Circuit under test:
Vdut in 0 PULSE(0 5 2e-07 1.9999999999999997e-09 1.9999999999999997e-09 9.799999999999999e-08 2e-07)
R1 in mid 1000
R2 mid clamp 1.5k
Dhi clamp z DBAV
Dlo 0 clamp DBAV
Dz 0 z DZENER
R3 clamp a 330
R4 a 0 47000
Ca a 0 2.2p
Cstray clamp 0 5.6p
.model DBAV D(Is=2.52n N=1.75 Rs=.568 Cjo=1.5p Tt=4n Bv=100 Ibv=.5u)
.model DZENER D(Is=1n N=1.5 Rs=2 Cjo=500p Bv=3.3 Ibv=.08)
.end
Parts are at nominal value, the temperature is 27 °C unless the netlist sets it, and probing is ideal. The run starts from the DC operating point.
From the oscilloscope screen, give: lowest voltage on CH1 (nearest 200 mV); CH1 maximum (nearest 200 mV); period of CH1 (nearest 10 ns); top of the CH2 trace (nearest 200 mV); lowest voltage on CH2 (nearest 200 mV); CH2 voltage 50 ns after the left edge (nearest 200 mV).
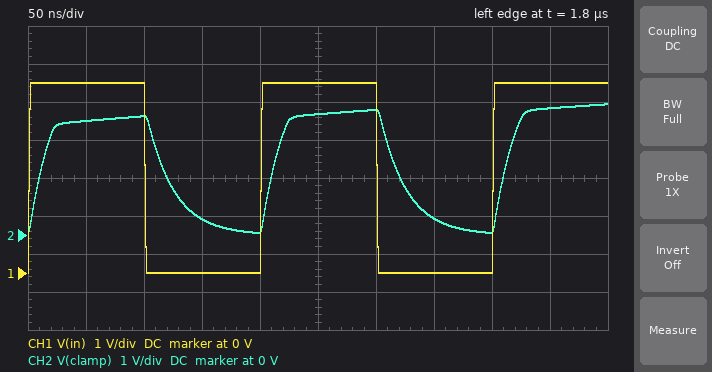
0 V
5.0 V
200 ns
3.4 V
0 V
3.0 V
